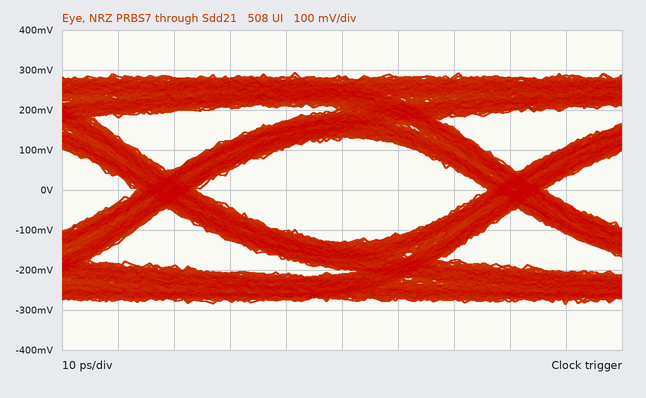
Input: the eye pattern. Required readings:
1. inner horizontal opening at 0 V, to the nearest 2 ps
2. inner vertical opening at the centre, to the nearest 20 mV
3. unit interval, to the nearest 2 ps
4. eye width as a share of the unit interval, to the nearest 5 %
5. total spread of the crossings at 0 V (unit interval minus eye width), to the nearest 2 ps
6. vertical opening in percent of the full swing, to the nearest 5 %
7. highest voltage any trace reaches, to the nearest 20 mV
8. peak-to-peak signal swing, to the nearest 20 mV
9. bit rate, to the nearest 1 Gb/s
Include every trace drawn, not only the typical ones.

52 ps
260 mV
62 ps
85 %
10 ps
45 %
300 mV
580 mV
16 Gb/s
